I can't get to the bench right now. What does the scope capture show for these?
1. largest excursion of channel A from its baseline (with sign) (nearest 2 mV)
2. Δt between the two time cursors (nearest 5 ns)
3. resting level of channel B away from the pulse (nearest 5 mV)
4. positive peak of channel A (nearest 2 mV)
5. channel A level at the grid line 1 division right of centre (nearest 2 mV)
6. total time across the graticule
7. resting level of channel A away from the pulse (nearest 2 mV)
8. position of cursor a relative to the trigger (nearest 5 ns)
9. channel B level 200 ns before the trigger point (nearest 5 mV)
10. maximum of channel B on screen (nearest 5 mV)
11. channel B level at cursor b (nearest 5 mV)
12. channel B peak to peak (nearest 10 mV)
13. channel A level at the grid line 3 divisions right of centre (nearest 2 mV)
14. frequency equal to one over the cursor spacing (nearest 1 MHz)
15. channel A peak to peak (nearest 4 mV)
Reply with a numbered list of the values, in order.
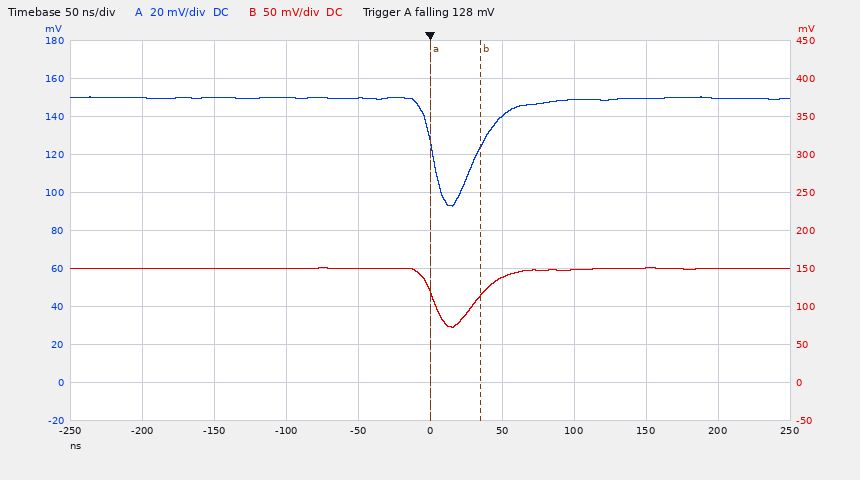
1. -56 mV
2. 35 ns
3. 150 mV
4. 150 mV
5. 140 mV
6. 500 ns
7. 150 mV
8. 0 ns
9. 150 mV
10. 150 mV
11. 115 mV
12. 80 mV
13. 150 mV
14. 29 MHz
15. 56 mV
